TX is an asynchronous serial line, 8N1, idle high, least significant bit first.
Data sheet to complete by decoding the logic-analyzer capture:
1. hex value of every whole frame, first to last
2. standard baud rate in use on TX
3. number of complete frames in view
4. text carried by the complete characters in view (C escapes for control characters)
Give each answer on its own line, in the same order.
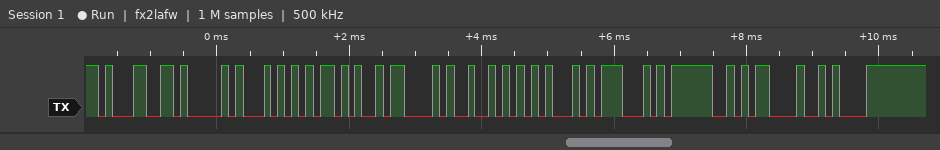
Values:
31 41 54 2B 43 52 45 47 3F 0D 0A
9600 baud
11
"1AT+CREG?\r\n"
